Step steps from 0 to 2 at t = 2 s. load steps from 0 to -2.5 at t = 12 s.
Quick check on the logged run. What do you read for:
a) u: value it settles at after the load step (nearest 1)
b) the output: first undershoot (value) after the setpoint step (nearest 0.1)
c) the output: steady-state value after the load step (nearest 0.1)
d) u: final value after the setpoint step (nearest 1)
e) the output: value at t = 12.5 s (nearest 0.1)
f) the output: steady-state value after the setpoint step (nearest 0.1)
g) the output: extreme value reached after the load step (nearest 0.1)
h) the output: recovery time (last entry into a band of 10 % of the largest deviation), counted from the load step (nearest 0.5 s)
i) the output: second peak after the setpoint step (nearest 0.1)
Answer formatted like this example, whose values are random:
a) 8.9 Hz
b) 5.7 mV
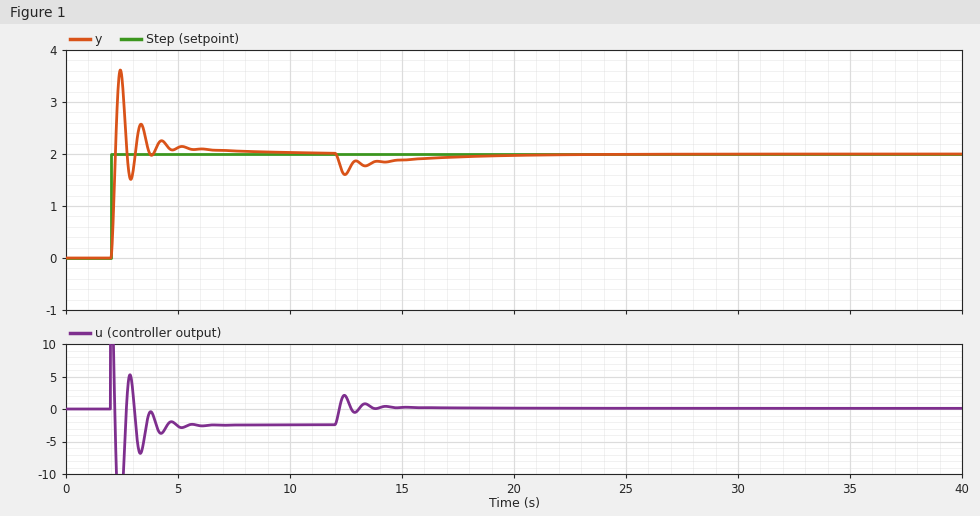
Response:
a) 0
b) 1.5
c) 2.0
d) -2
e) 1.6
f) 2.0
g) 1.6
h) 6.5 s
i) 2.6
